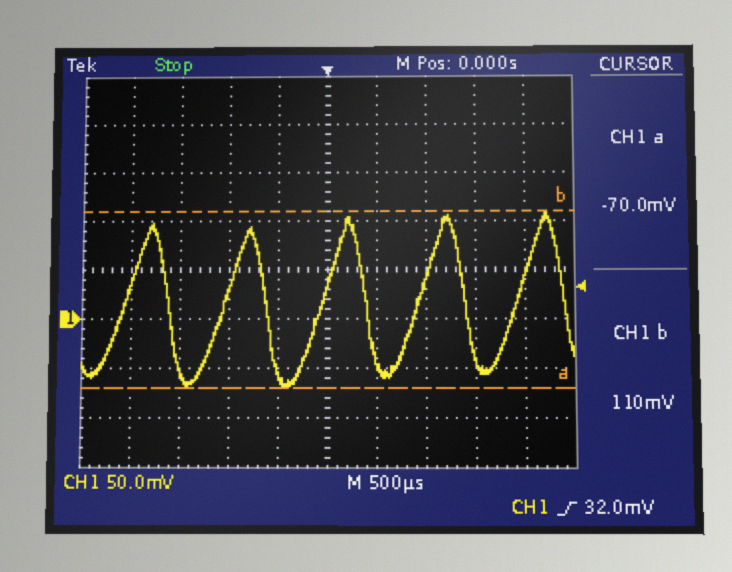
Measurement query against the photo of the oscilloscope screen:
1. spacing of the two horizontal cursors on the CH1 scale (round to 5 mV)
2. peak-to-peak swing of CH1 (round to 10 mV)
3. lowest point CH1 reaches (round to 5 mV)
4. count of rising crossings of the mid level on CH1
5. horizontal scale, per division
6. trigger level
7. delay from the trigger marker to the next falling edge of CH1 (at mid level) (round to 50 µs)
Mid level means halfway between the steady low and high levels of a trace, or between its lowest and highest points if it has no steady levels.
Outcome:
180 mV
180 mV
-70 mV
5
500 µs
32.0 mV
400 µs
